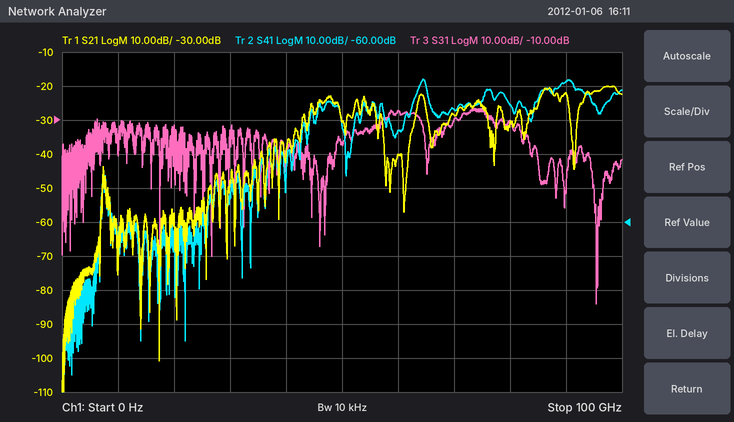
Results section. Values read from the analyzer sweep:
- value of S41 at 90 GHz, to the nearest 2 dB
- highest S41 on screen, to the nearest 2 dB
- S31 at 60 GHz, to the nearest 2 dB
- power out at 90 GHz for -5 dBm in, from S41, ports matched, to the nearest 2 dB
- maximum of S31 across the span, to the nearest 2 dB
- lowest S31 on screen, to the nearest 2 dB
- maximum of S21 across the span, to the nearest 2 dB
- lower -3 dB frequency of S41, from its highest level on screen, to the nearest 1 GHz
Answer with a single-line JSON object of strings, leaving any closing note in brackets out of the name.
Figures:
{"value of S41 at 90 GHz, to the nearest 2 dB": "-18 dB", "highest S41 on screen, to the nearest 2 dB": "-18 dB", "S31 at 60 GHz, to the nearest 2 dB": "-8 dB", "power out at 90 GHz for -5 dBm in, from S41, ports matched, to the nearest 2 dB": "-24 dBm", "maximum of S31 across the span, to the nearest 2 dB": "-6 dB", "lowest S31 on screen, to the nearest 2 dB": "-64 dB", "maximum of S21 across the span, to the nearest 2 dB": "-20 dB", "lower -3 dB frequency of S41, from its highest level on screen, to the nearest 1 GHz": "64 GHz"}
